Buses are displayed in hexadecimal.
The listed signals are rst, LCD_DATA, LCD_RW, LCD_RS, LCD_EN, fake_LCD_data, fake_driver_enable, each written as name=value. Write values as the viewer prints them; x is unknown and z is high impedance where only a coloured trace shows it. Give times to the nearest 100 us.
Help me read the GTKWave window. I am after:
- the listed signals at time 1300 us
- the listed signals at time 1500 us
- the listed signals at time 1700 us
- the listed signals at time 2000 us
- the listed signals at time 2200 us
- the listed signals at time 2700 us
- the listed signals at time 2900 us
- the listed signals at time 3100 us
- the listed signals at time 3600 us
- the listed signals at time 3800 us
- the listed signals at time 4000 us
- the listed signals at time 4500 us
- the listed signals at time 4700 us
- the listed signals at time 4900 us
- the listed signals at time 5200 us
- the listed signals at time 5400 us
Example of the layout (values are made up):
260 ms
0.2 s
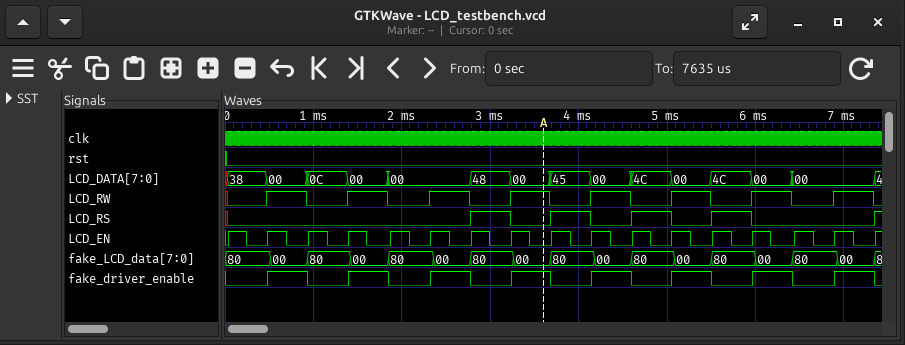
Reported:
rst=0, LCD_DATA=0C, LCD_RW=0, LCD_RS=0, LCD_EN=0, fake_LCD_data=80, fake_driver_enable=0
rst=0, LCD_DATA=00, LCD_RW=1, LCD_RS=0, LCD_EN=1, fake_LCD_data=00, fake_driver_enable=1
rst=0, LCD_DATA=00, LCD_RW=1, LCD_RS=0, LCD_EN=0, fake_LCD_data=00, fake_driver_enable=1
rst=0, LCD_DATA=00, LCD_RW=0, LCD_RS=0, LCD_EN=1, fake_LCD_data=80, fake_driver_enable=0
rst=0, LCD_DATA=00, LCD_RW=0, LCD_RS=0, LCD_EN=0, fake_LCD_data=80, fake_driver_enable=0
rst=0, LCD_DATA=00, LCD_RW=1, LCD_RS=0, LCD_EN=0, fake_LCD_data=00, fake_driver_enable=1
rst=0, LCD_DATA=48, LCD_RW=0, LCD_RS=1, LCD_EN=1, fake_LCD_data=80, fake_driver_enable=0
rst=0, LCD_DATA=48, LCD_RW=0, LCD_RS=1, LCD_EN=0, fake_LCD_data=80, fake_driver_enable=0
rst=0, LCD_DATA=00, LCD_RW=1, LCD_RS=0, LCD_EN=0, fake_LCD_data=00, fake_driver_enable=1
rst=0, LCD_DATA=45, LCD_RW=0, LCD_RS=1, LCD_EN=1, fake_LCD_data=80, fake_driver_enable=0
rst=0, LCD_DATA=45, LCD_RW=0, LCD_RS=1, LCD_EN=0, fake_LCD_data=80, fake_driver_enable=0
rst=0, LCD_DATA=00, LCD_RW=1, LCD_RS=0, LCD_EN=0, fake_LCD_data=00, fake_driver_enable=1
rst=0, LCD_DATA=4C, LCD_RW=0, LCD_RS=1, LCD_EN=1, fake_LCD_data=80, fake_driver_enable=0
rst=0, LCD_DATA=4C, LCD_RW=0, LCD_RS=1, LCD_EN=0, fake_LCD_data=80, fake_driver_enable=0
rst=0, LCD_DATA=00, LCD_RW=1, LCD_RS=0, LCD_EN=1, fake_LCD_data=00, fake_driver_enable=1
rst=0, LCD_DATA=00, LCD_RW=1, LCD_RS=0, LCD_EN=0, fake_LCD_data=00, fake_driver_enable=1
